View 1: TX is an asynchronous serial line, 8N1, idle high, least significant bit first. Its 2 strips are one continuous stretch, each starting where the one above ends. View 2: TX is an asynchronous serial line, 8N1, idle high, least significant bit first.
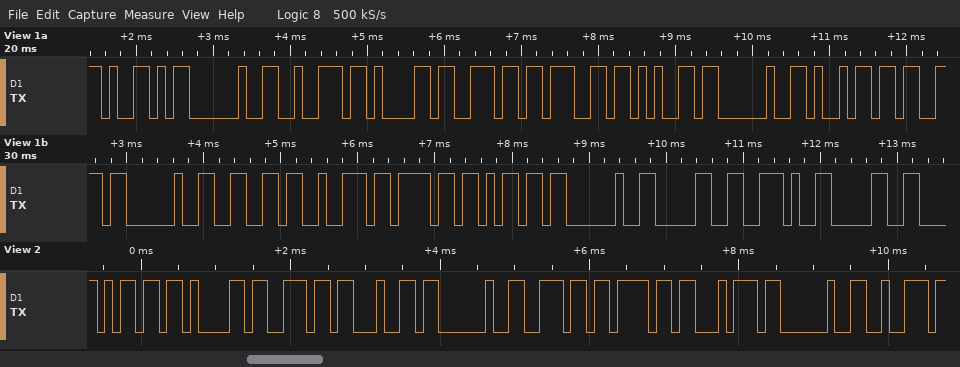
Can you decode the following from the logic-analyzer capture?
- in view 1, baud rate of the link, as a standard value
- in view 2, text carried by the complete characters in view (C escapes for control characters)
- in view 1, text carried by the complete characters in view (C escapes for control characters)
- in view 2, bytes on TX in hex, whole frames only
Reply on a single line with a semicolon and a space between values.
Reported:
9600 baud; "mand not r"; "Y range is from 0.0"; 6D 61 6E 64 20 6E 6F 74 20 72
